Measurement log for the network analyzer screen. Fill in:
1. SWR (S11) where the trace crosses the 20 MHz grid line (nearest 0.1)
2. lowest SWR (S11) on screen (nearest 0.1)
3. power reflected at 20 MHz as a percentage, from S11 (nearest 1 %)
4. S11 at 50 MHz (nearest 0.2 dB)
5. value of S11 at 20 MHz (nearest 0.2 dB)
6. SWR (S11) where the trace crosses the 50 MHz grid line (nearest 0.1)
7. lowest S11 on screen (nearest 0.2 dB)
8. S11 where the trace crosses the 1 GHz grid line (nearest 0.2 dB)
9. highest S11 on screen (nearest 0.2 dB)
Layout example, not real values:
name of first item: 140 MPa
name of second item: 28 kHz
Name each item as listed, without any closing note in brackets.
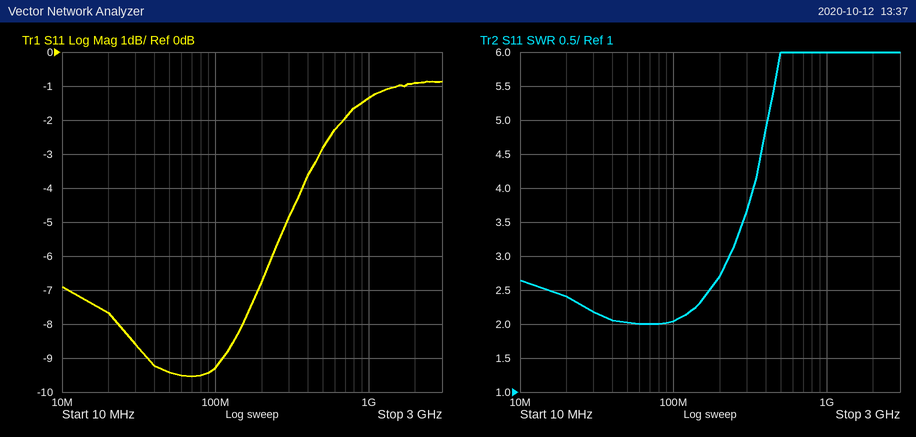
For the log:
SWR (S11) where the trace crosses the 20 MHz grid line: 2.4
lowest SWR (S11) on screen: 2.0
power reflected at 20 MHz as a percentage, from S11: 17 %
S11 at 50 MHz: -9.4 dB
value of S11 at 20 MHz: -7.6 dB
SWR (S11) where the trace crosses the 50 MHz grid line: 2.0
lowest S11 on screen: -9.6 dB
S11 where the trace crosses the 1 GHz grid line: -1.4 dB
highest S11 on screen: -0.8 dB
